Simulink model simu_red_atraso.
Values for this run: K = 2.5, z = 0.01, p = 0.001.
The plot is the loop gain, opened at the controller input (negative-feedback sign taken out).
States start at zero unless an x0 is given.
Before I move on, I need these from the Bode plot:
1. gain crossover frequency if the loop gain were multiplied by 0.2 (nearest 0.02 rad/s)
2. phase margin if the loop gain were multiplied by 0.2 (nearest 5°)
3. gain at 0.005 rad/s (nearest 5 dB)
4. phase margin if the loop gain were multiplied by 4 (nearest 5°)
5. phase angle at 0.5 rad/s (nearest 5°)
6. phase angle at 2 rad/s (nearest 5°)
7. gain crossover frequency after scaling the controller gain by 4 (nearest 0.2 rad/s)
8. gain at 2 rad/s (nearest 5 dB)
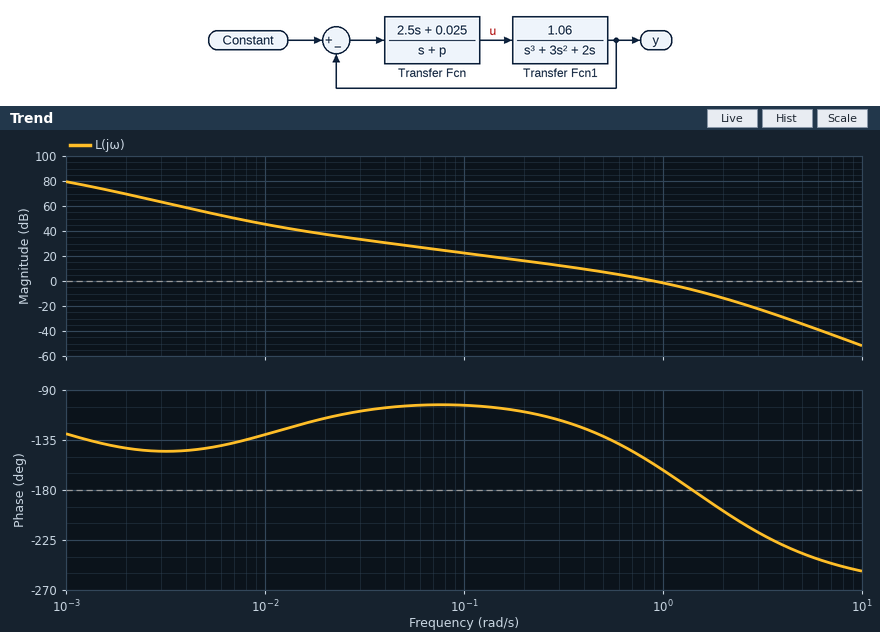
0.26 rad/s
65°
55 dB
-15°
-130°
-200°
1.8 rad/s
-15 dB
